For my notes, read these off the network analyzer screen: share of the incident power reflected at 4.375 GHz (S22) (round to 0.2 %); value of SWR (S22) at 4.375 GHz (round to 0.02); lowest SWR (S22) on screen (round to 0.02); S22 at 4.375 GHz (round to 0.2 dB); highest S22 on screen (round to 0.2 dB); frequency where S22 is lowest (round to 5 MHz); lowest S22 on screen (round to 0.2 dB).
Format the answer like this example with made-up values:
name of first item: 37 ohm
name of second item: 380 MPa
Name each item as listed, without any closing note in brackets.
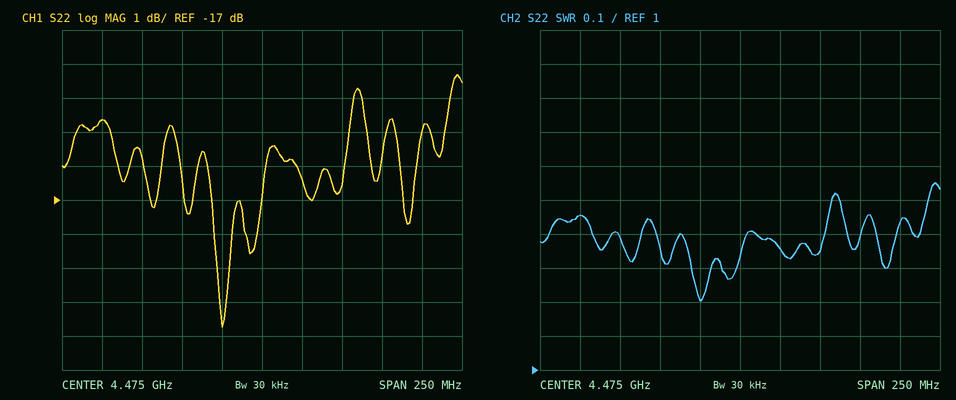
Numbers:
share of the incident power reflected at 4.375 GHz (S22): 3.4 %
value of SWR (S22) at 4.375 GHz: 1.46
lowest SWR (S22) on screen: 1.20
S22 at 4.375 GHz: -14.6 dB
highest S22 on screen: -13.4 dB
frequency where S22 is lowest: 4.450 GHz
lowest S22 on screen: -20.8 dB
